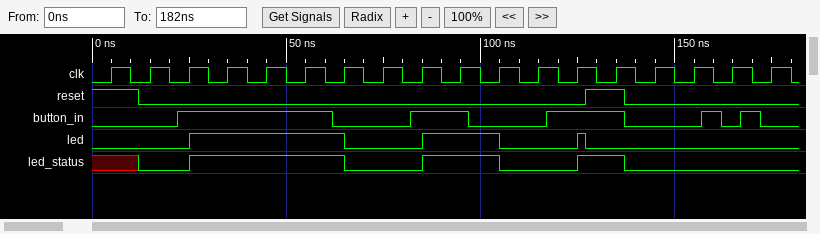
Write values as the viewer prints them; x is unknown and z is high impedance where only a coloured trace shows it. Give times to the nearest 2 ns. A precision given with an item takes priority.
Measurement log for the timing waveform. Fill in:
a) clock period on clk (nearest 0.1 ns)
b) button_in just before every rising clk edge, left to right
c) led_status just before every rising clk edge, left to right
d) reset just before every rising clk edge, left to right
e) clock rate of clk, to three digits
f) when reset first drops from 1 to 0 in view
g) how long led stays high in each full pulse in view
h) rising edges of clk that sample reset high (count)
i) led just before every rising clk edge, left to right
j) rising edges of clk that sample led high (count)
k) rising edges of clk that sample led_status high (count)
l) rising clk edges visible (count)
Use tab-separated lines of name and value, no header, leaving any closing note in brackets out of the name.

clock period on clk	10 ns
button_in just before every rising clk edge, left to right	0 0 1 1 1 1 0 0 1 1 0 0 1 1 0 0 0 0
led_status just before every rising clk edge, left to right	x 0 0 1 1 1 1 0 0 1 1 0 0 1 0 0 0 0
reset just before every rising clk edge, left to right	1 0 0 0 0 0 0 0 0 0 0 0 0 1 0 0 0 0
clock rate of clk, to three digits	100 MHz
when reset first drops from 1 to 0 in view	12 ns
how long led stays high in each full pulse in view	40 ns, 20 ns, 2 ns
rising edges of clk that sample reset high	2
led just before every rising clk edge, left to right	0 0 0 1 1 1 1 0 0 1 1 0 0 0 0 0 0 0
rising edges of clk that sample led high	6
rising edges of clk that sample led_status high	7
rising clk edges visible	18
